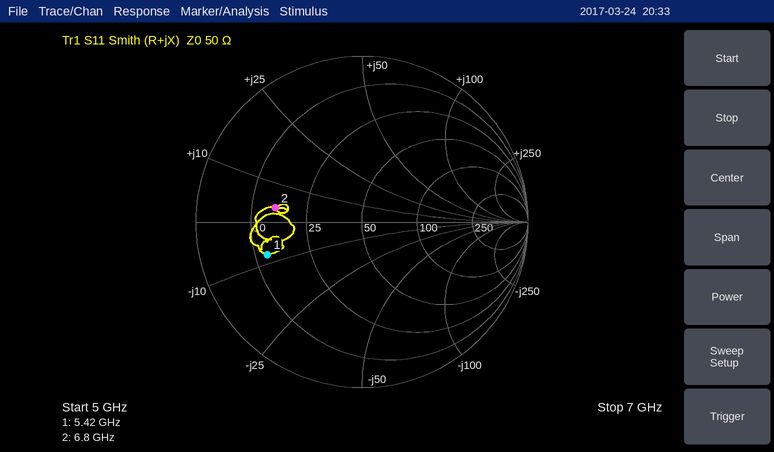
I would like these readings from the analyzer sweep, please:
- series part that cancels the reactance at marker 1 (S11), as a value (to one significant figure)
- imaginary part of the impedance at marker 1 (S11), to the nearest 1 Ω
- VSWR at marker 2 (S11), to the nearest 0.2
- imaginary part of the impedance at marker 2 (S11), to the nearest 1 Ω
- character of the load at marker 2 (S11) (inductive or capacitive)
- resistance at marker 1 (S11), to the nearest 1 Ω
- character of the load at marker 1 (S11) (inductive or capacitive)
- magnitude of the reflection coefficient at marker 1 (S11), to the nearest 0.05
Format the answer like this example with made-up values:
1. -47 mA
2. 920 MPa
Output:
1. 200 pH
2. -8 Ω
3. 3.2
4. +4 Ω
5. inductive
6. 13 Ω
7. capacitive
8. 0.60
